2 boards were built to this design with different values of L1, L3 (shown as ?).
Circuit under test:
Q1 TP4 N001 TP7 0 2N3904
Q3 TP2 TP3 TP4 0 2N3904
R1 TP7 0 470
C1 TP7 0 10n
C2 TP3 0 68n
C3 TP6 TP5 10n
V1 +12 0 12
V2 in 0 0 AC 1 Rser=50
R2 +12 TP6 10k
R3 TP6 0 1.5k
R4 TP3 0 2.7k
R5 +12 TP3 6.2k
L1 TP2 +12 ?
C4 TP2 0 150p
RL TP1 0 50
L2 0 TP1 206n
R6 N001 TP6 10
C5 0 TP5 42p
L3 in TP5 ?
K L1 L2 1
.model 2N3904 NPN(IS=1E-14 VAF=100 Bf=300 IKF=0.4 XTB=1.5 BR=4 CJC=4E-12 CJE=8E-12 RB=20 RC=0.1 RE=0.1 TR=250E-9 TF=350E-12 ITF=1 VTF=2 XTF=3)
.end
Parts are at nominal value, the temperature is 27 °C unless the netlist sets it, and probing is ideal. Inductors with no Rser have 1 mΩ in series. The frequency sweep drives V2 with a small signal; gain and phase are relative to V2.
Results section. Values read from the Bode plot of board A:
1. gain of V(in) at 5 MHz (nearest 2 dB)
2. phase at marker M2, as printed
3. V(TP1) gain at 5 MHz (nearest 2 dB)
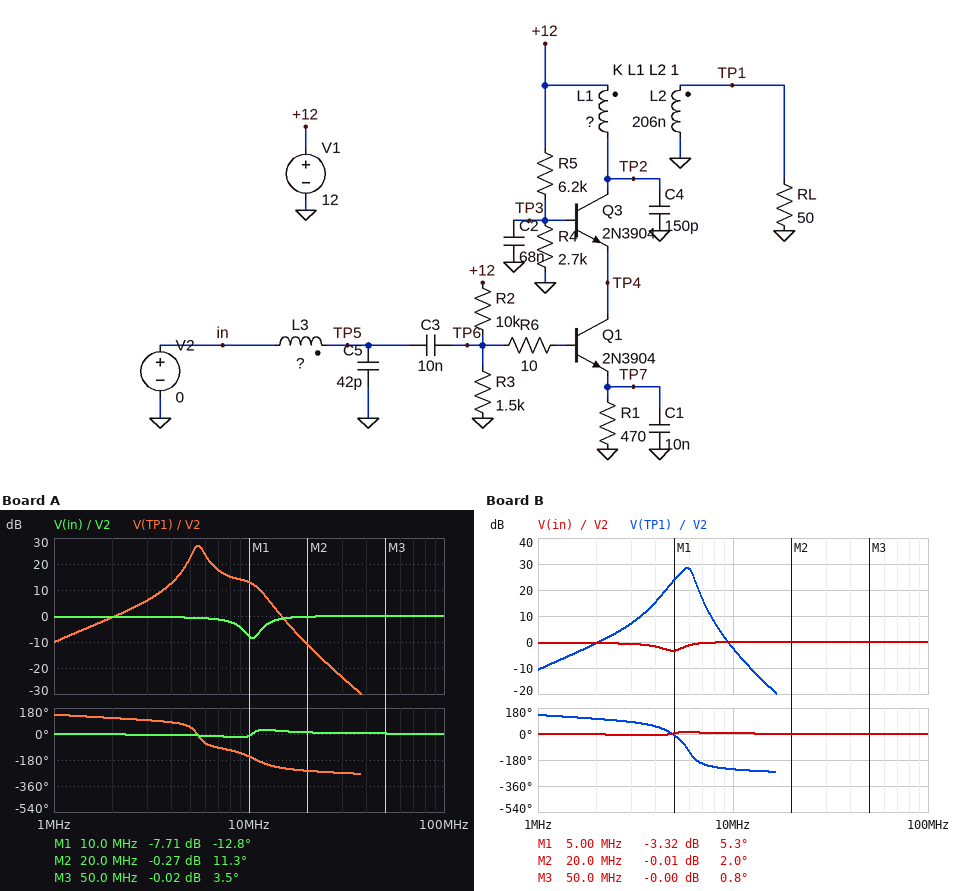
0 dB
11.3 deg
22 dB
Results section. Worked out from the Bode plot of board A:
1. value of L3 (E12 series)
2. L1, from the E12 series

2.7 µH
5.6 µH
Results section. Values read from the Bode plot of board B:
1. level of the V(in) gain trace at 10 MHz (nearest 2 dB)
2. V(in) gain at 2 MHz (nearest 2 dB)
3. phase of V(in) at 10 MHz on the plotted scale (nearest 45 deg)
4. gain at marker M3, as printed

0 dB
0 dB
0 deg
-0.00 dB
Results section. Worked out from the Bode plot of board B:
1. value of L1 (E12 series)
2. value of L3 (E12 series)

4.7 µH
12 µH
